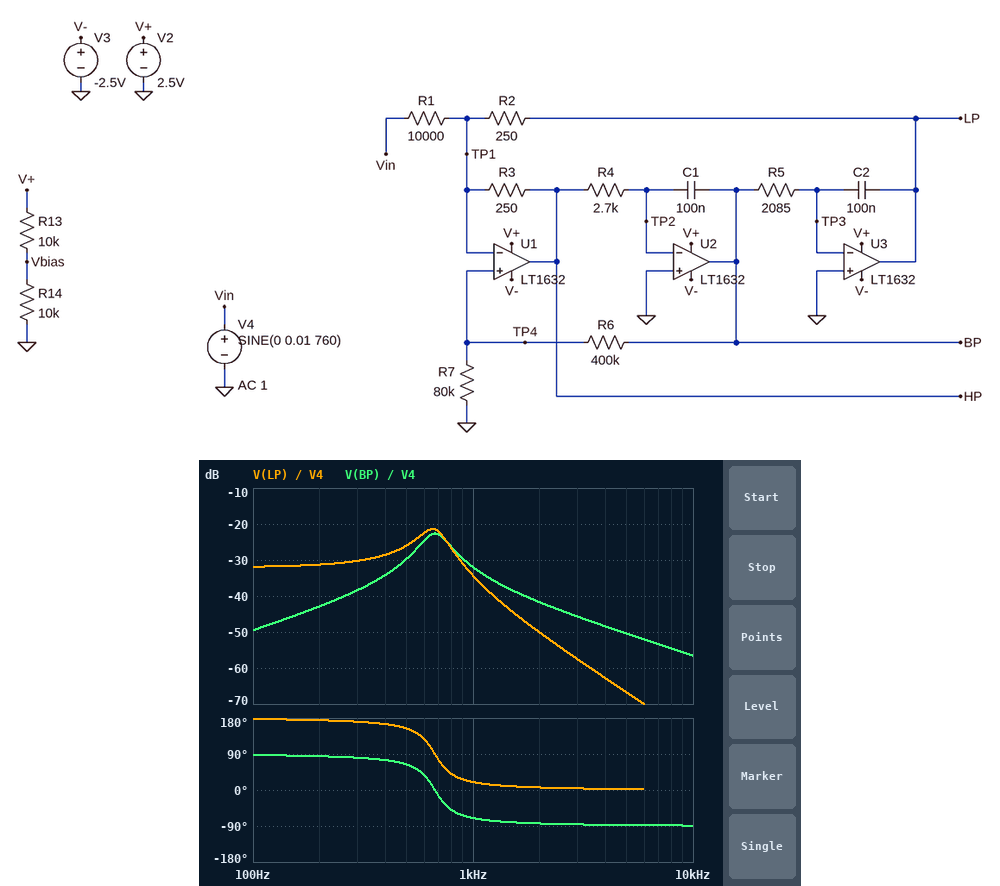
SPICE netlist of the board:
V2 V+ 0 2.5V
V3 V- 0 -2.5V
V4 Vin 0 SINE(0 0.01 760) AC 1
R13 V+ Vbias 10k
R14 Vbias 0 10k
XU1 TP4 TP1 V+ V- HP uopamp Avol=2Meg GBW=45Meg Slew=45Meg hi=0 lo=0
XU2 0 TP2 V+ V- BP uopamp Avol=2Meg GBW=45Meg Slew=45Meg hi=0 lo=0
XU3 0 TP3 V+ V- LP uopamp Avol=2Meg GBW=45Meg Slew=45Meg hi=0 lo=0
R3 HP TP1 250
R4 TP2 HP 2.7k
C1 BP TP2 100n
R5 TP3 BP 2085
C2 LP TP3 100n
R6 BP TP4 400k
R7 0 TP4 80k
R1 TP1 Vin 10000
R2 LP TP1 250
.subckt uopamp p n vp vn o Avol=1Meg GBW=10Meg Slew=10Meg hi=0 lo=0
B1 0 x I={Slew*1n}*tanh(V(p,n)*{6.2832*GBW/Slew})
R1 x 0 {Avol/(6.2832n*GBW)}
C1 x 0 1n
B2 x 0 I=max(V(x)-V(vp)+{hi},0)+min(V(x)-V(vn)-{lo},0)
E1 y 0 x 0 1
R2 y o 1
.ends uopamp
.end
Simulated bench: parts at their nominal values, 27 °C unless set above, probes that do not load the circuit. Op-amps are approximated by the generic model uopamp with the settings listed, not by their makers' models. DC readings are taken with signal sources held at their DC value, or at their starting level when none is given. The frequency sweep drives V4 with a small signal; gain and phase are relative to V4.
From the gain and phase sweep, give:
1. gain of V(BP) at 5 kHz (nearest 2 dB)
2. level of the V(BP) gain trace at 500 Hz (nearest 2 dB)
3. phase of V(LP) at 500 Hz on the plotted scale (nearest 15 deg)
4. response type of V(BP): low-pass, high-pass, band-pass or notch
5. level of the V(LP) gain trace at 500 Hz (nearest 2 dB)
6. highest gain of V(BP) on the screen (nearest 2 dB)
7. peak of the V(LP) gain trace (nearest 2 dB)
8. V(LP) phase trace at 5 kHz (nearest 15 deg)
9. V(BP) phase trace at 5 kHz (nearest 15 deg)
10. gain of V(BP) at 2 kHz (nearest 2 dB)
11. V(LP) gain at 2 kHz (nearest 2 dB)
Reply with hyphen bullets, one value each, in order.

- -50 dB
- -30 dB
- 150 deg
- band-pass
- -26 dB
- -22 dB
- -22 dB
- 0 deg
- -90 deg
- -42 dB
- -50 dB
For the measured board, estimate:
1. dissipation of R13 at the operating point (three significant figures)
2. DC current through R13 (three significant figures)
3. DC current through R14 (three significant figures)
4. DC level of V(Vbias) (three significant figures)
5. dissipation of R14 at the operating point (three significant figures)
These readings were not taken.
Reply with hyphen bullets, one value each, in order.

- 156 µW
- 125 µA
- 125 µA
- 1.25 V
- 156 µW
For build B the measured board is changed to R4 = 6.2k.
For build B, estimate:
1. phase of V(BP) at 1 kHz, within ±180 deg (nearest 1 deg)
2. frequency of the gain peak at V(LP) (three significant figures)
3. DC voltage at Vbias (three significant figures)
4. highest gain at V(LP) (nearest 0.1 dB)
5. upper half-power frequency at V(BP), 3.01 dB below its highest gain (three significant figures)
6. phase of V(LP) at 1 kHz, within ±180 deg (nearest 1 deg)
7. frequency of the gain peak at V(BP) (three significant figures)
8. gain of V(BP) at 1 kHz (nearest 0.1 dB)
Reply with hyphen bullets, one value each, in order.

- -84 deg
- 438 Hz
- 1.25 V
- -17.8 dB
- 488 Hz
- 6 deg
- 443 Hz
- -42.0 dB
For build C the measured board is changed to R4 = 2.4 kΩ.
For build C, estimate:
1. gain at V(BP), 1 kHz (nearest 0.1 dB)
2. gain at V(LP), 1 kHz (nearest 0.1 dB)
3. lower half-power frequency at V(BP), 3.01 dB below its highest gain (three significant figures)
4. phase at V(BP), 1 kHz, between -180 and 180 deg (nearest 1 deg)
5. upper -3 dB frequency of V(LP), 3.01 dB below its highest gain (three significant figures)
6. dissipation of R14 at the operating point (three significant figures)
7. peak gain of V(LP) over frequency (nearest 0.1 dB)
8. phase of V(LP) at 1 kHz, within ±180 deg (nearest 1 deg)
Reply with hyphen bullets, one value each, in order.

- -30.3 dB
- -32.6 dB
- 608 Hz
- -66 deg
- 799 Hz
- 156 µW
- -21.9 dB
- 24 deg
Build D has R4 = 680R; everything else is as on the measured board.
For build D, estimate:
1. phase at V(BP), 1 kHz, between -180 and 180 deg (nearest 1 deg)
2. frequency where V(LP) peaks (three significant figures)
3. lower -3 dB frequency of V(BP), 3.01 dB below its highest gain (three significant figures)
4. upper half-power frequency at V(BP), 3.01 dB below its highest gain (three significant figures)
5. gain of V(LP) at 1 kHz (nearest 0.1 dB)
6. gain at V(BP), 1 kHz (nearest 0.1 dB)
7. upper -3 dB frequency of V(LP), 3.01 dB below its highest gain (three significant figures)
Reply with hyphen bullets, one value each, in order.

- 45 deg
- 1.21 kHz
- 999 Hz
- 1.79 kHz
- -27.9 dB
- -25.6 dB
- 1.58 kHz
